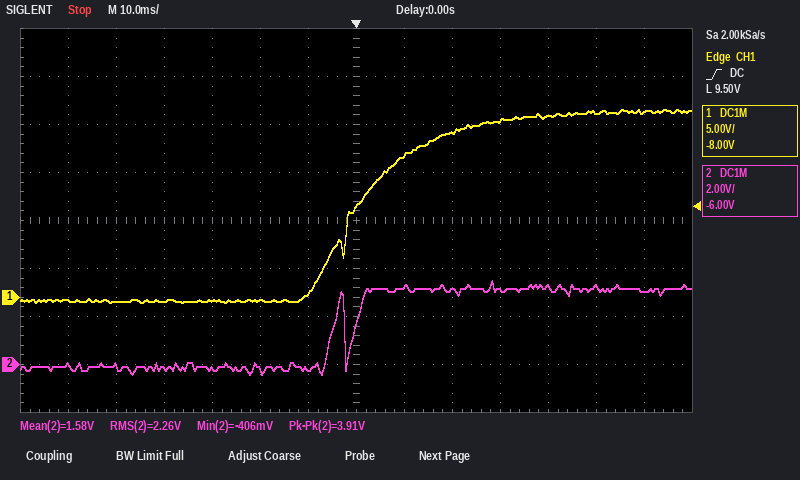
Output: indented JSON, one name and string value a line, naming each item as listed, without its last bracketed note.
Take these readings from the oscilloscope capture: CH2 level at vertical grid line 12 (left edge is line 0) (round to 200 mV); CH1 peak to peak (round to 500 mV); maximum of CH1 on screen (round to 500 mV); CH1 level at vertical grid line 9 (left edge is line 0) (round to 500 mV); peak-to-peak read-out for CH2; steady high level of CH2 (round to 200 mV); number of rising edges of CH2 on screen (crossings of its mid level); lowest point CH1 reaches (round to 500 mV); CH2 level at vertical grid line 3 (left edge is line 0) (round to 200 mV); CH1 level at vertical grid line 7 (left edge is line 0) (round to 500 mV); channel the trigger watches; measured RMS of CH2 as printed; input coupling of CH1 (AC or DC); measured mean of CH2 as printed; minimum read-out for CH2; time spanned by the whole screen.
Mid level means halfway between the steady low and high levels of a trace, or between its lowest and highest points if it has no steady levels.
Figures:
{
  "CH2 level at vertical grid line 12 (left edge is line 0)": "3.2 V",
  "CH1 peak to peak": "20.0 V",
  "maximum of CH1 on screen": "19.5 V",
  "CH1 level at vertical grid line 9 (left edge is line 0)": "17.0 V",
  "peak-to-peak read-out for CH2": "3.91 V",
  "steady high level of CH2": "3.2 V",
  "number of rising edges of CH2 on screen": "2",
  "lowest point CH1 reaches": "-500 mV",
  "CH2 level at vertical grid line 3 (left edge is line 0)": "-200 mV",
  "CH1 level at vertical grid line 7 (left edge is line 0)": "9.5 V",
  "channel the trigger watches": "CH1",
  "measured RMS of CH2 as printed": "2.26 V",
  "input coupling of CH1": "DC",
  "measured mean of CH2 as printed": "1.58 V",
  "minimum read-out for CH2": "-406 mV",
  "time spanned by the whole screen": "140 ms"
}
